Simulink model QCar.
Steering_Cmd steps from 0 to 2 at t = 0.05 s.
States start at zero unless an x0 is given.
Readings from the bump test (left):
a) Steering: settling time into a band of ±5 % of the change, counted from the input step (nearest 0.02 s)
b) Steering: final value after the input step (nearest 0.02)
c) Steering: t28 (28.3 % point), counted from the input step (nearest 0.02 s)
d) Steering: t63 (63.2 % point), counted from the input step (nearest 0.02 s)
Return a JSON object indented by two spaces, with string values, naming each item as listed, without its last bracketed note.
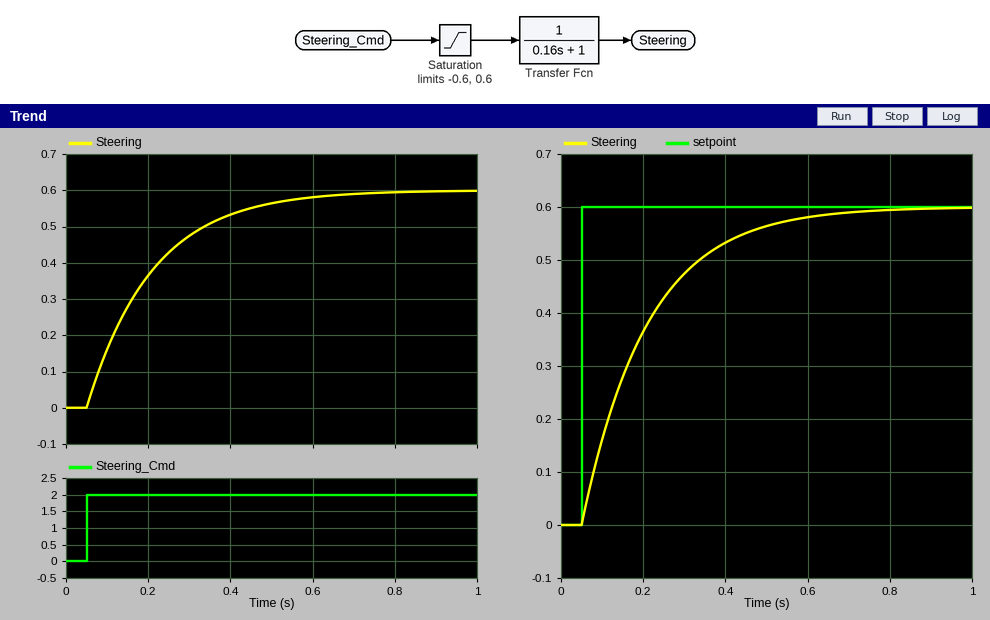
{
  "Steering: settling time into a band of ±5 % of the change, counted from the input step": "0.48 s",
  "Steering: final value after the input step": "0.60",
  "Steering: t28 (28.3 % point), counted from the input step": "0.06 s",
  "Steering: t63 (63.2 % point), counted from the input step": "0.16 s"
}
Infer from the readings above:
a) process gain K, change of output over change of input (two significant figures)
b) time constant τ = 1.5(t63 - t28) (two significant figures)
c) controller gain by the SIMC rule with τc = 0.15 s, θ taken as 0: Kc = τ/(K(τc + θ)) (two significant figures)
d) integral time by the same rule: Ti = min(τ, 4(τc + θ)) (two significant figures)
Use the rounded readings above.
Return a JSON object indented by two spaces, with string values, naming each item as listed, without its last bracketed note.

{
  "process gain K, change of output over change of input": "0.30",
  "time constant τ = 1.5(t63 - t28)": "0.15 s",
  "controller gain by the SIMC rule with τc = 0.15 s, θ taken as 0: Kc = τ/(K(τc + θ))": "3.3",
  "integral time by the same rule: Ti = min(τ, 4(τc + θ))": "0.15 s"
}
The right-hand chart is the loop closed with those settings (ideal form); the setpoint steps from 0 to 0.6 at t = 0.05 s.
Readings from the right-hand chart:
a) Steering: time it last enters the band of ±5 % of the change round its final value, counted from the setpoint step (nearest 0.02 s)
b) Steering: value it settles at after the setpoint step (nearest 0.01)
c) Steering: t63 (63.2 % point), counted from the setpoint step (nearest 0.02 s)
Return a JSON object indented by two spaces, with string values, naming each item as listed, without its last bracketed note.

{
  "Steering: time it last enters the band of ±5 % of the change round its final value, counted from the setpoint step": "0.48 s",
  "Steering: value it settles at after the setpoint step": "0.60",
  "Steering: t63 (63.2 % point), counted from the setpoint step": "0.16 s"
}
